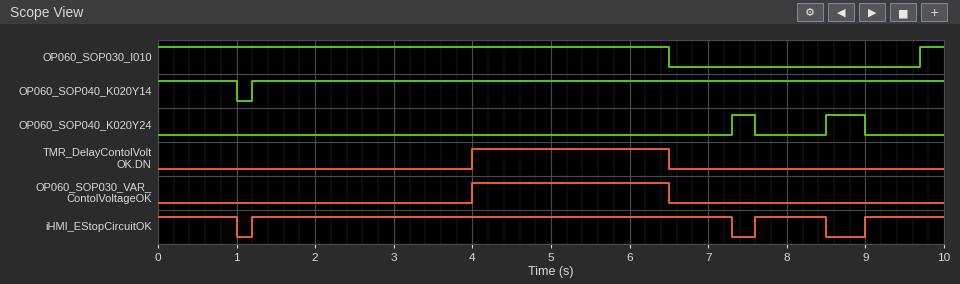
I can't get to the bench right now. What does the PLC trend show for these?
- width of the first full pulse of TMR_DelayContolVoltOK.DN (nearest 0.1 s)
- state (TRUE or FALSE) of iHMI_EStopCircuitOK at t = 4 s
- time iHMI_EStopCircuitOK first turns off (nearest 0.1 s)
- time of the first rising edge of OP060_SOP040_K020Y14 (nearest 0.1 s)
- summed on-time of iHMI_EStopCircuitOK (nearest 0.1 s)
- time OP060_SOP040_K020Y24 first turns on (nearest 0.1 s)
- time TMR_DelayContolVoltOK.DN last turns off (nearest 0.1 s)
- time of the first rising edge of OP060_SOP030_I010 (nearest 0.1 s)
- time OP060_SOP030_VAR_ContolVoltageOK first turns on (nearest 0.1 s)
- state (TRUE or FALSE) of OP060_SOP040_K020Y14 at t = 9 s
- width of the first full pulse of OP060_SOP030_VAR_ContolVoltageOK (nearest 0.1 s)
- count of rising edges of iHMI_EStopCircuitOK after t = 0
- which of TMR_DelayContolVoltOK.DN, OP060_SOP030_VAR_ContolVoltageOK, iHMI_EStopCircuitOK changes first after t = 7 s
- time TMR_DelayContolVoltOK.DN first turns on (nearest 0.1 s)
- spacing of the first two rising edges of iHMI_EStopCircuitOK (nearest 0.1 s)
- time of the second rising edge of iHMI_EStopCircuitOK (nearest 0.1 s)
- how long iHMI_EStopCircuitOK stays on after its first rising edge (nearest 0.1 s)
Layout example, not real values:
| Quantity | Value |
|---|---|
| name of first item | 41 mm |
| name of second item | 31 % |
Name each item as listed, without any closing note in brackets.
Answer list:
| Quantity | Value |
|---|---|
| width of the first full pulse of TMR_DelayContolVoltOK.DN | 2.5 s |
| state (TRUE or FALSE) of iHMI_EStopCircuitOK at t = 4 s | TRUE |
| time iHMI_EStopCircuitOK first turns off | 1.0 s |
| time of the first rising edge of OP060_SOP040_K020Y14 | 1.2 s |
| summed on-time of iHMI_EStopCircuitOK | 9.0 s |
| time OP060_SOP040_K020Y24 first turns on | 7.3 s |
| time TMR_DelayContolVoltOK.DN last turns off | 6.5 s |
| time of the first rising edge of OP060_SOP030_I010 | 9.7 s |
| time OP060_SOP030_VAR_ContolVoltageOK first turns on | 4.0 s |
| state (TRUE or FALSE) of OP060_SOP040_K020Y14 at t = 9 s | TRUE |
| width of the first full pulse of OP060_SOP030_VAR_ContolVoltageOK | 2.5 s |
| count of rising edges of iHMI_EStopCircuitOK after t = 0 | 3 |
| which of TMR_DelayContolVoltOK.DN, OP060_SOP030_VAR_ContolVoltageOK, iHMI_EStopCircuitOK changes first after t = 7 s | iHMI_EStopCircuitOK |
| time TMR_DelayContolVoltOK.DN first turns on | 4.0 s |
| spacing of the first two rising edges of iHMI_EStopCircuitOK | 6.4 s |
| time of the second rising edge of iHMI_EStopCircuitOK | 7.6 s |
| how long iHMI_EStopCircuitOK stays on after its first rising edge | 6.1 s |
